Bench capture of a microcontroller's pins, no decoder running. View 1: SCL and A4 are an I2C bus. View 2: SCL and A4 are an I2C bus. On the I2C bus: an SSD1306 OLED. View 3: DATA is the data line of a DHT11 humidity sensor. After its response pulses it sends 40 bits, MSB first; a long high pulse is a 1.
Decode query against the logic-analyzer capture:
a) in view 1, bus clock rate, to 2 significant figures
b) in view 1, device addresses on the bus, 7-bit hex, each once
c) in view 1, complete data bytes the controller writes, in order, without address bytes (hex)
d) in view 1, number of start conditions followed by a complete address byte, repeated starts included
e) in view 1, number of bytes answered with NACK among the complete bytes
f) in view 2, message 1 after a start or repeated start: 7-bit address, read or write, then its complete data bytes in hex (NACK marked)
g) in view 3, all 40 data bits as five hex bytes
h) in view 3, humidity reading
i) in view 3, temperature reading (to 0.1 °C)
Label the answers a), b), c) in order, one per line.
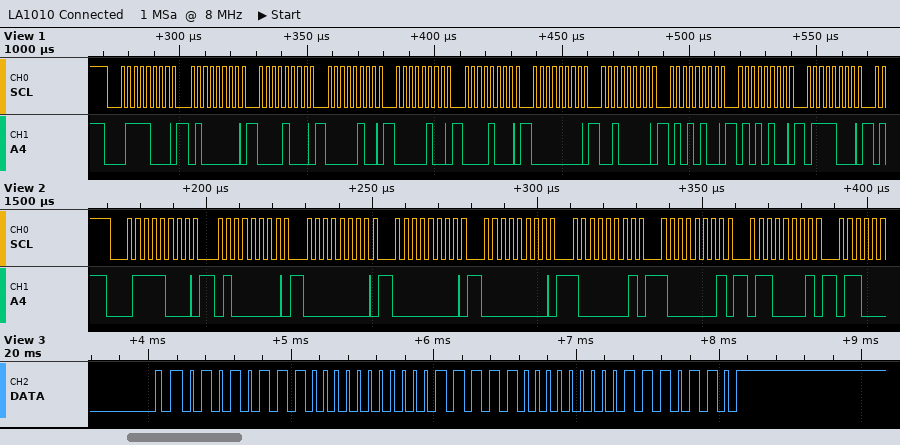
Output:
a) 400 kHz
b) 0x3C
c) 40 08 04 04 08 00 20 54 54 78
d) 1
e) 0
f) 0x3C write: 40 00 00 00 81 81 61
g) 57 00 1F 00 76
h) 87 %
i) 31.0 °C
